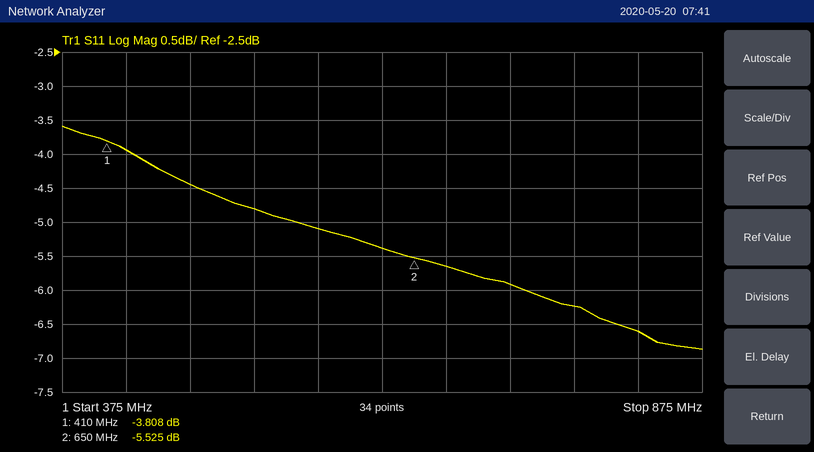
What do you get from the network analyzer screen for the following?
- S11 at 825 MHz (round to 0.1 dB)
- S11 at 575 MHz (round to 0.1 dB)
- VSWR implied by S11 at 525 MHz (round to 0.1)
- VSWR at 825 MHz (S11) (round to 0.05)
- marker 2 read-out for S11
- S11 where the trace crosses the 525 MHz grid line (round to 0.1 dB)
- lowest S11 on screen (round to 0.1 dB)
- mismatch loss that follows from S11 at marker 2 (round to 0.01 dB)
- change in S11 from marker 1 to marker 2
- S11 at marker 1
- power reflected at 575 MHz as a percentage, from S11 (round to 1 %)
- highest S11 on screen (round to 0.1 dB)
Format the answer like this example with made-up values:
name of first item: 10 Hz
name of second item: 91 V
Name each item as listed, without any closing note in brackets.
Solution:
S11 at 825 MHz: -6.6 dB
S11 at 575 MHz: -5.1 dB
VSWR implied by S11 at 525 MHz: 3.7
VSWR at 825 MHz (S11): 2.75
marker 2 read-out for S11: -5.525 dB
S11 where the trace crosses the 525 MHz grid line: -4.8 dB
lowest S11 on screen: -6.9 dB
mismatch loss that follows from S11 at marker 2: 1.43 dB
change in S11 from marker 1 to marker 2: -1.717 dB
S11 at marker 1: -3.808 dB
power reflected at 575 MHz as a percentage, from S11: 31 %
highest S11 on screen: -3.6 dB
